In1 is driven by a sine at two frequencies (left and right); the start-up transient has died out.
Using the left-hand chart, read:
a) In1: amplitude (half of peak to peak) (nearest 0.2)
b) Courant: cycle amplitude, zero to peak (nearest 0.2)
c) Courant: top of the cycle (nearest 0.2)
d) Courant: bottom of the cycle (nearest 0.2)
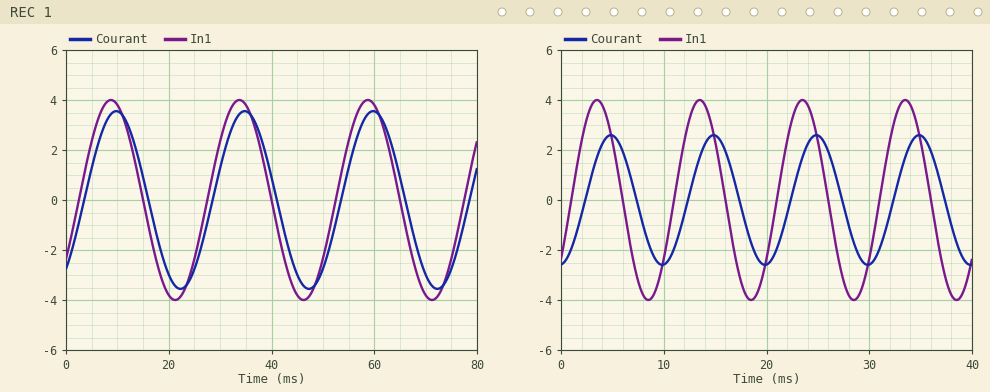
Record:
4.0
3.6
3.6
-3.6
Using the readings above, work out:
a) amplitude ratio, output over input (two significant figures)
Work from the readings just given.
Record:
0.90
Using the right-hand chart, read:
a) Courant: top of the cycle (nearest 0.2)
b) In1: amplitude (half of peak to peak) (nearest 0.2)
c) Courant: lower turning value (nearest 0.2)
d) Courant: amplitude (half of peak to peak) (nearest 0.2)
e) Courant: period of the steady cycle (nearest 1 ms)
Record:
2.6
4.0
-2.6
2.6
10 ms
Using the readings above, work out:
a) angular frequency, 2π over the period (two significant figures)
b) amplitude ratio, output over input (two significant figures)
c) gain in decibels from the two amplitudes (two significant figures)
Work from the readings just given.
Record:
0.63 rad/ms
0.65
-3.7 dB
